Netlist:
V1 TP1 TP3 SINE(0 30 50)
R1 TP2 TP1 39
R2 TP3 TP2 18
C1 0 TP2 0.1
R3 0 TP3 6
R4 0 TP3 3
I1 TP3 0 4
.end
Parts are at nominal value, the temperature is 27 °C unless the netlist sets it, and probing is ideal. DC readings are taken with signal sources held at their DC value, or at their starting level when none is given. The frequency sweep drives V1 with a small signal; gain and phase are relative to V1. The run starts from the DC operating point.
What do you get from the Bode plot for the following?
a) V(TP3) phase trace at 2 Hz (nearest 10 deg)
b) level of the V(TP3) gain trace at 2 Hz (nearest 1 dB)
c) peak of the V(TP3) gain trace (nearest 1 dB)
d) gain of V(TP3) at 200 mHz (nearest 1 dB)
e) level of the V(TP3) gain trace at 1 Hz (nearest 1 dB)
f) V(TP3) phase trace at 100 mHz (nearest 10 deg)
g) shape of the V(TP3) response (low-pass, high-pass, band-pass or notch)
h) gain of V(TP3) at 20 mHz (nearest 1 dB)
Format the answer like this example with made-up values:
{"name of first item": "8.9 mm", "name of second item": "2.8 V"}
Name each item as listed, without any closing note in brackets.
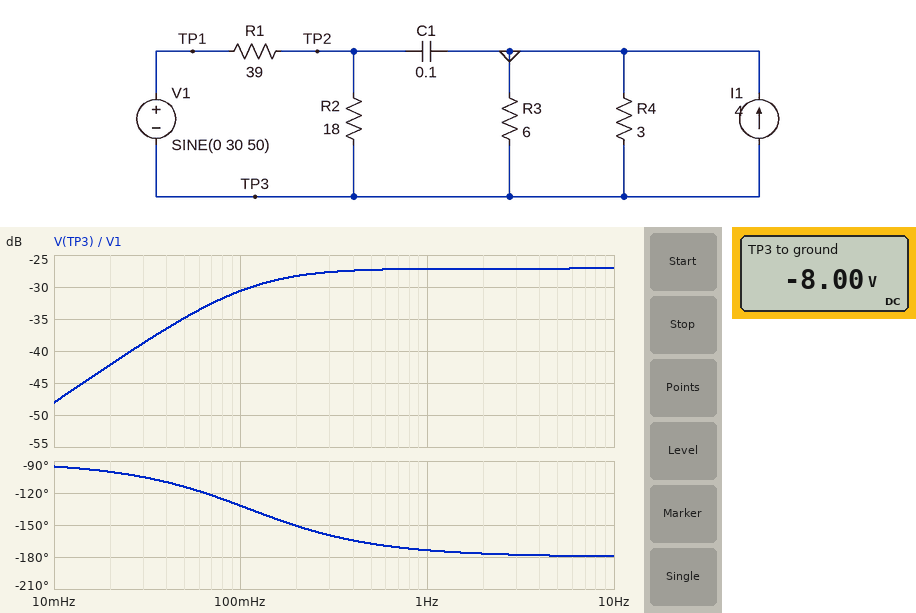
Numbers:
{"V(TP3) phase trace at 2 Hz": "-180 deg", "level of the V(TP3) gain trace at 2 Hz": "-27 dB", "peak of the V(TP3) gain trace": "-27 dB", "gain of V(TP3) at 200 mHz": "-28 dB", "level of the V(TP3) gain trace at 1 Hz": "-27 dB", "V(TP3) phase trace at 100 mHz": "-130 deg", "shape of the V(TP3) response": "high-pass", "gain of V(TP3) at 20 mHz": "-42 dB"}
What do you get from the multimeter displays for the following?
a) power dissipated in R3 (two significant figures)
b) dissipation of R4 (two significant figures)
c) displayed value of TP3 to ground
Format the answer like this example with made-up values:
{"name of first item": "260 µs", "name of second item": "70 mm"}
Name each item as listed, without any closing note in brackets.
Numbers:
{"power dissipated in R3": "11 W", "dissipation of R4": "21 W", "displayed value of TP3 to ground": "-8.00 V"}
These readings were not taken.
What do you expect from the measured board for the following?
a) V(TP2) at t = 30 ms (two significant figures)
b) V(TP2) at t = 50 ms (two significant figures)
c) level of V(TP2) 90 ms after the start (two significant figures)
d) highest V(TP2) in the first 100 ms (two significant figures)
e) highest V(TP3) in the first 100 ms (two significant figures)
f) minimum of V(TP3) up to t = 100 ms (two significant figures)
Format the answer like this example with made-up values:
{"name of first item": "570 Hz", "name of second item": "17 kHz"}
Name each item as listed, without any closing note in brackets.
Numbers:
{"V(TP2) at t = 30 ms": "-8.0 V", "V(TP2) at t = 50 ms": "-8.0 V", "level of V(TP2) 90 ms after the start": "-8.0 V", "highest V(TP2) in the first 100 ms": "-8.0 V", "highest V(TP3) in the first 100 ms": "-6.7 V", "minimum of V(TP3) up to t = 100 ms": "-9.3 V"}
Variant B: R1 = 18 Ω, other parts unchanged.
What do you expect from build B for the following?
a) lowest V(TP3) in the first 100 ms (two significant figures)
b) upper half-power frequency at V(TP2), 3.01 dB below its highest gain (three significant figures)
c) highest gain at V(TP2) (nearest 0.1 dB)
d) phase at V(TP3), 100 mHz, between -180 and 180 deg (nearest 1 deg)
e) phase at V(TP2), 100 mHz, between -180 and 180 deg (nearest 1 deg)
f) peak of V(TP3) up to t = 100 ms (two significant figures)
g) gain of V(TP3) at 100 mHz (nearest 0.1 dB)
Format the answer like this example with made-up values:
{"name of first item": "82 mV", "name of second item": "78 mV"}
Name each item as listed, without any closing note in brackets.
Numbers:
{"lowest V(TP3) in the first 100 ms": "-11 V", "upper half-power frequency at V(TP2), 3.01 dB below its highest gain": "145 mHz", "highest gain at V(TP2)": "-6.0 dB", "phase at V(TP3), 100 mHz, between -180 and 180 deg": "-125 deg", "phase at V(TP2), 100 mHz, between -180 and 180 deg": "-35 deg", "peak of V(TP3) up to t = 100 ms": "-5.3 V", "gain of V(TP3) at 100 mHz": "-25.7 dB"}
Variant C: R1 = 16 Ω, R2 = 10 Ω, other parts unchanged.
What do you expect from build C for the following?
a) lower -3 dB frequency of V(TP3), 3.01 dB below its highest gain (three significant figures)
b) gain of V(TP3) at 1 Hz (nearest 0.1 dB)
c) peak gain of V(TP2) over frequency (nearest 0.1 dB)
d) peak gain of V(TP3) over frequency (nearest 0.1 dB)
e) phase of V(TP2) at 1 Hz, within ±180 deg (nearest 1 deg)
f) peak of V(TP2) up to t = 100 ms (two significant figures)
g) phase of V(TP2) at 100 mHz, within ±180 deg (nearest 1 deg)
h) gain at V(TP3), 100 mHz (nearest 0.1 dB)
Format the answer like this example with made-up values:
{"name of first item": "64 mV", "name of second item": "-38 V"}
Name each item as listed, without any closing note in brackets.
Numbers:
{"lower -3 dB frequency of V(TP3), 3.01 dB below its highest gain": "195 mHz", "gain of V(TP3) at 1 Hz": "-20.7 dB", "peak gain of V(TP2) over frequency": "-8.3 dB", "peak gain of V(TP3) over frequency": "-20.5 dB", "phase of V(TP2) at 1 Hz, within ±180 deg": "-79 deg", "peak of V(TP2) up to t = 100 ms": "-7.9 V", "phase of V(TP2) at 100 mHz, within ±180 deg": "-27 deg", "gain at V(TP3), 100 mHz": "-27.3 dB"}
